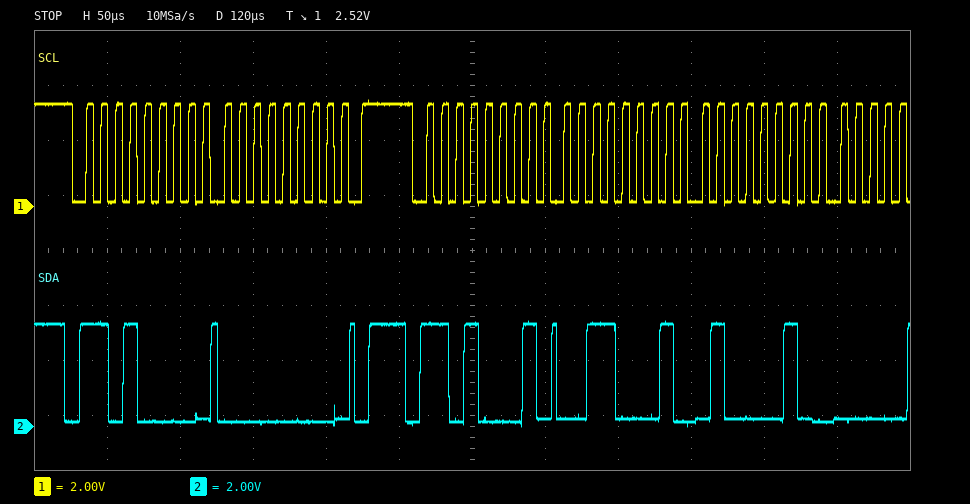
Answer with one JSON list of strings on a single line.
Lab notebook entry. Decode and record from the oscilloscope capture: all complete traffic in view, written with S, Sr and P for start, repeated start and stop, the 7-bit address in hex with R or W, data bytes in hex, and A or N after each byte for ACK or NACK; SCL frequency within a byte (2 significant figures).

["S 68W A 00 A P S 68R A 31 A 42 A", "100 kHz"]
